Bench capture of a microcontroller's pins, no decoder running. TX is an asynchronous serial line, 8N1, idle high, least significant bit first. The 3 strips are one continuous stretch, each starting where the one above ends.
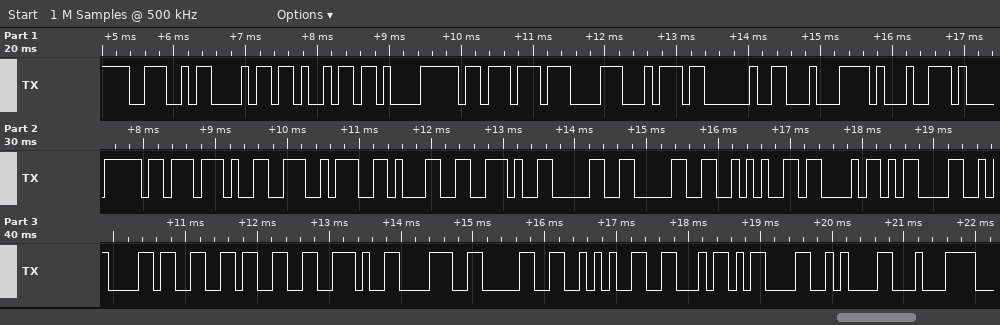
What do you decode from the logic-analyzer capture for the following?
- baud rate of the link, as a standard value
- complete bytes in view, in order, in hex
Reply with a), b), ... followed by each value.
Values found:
a) 9600 baud
b) 4E 68 69 E1 BB 87 74 20 C4 91 E1 BB 99 3A 31 2E 30 30 2A 43 0D 0A 33 33 2E 38 30 2A 46 0D 0A C4
